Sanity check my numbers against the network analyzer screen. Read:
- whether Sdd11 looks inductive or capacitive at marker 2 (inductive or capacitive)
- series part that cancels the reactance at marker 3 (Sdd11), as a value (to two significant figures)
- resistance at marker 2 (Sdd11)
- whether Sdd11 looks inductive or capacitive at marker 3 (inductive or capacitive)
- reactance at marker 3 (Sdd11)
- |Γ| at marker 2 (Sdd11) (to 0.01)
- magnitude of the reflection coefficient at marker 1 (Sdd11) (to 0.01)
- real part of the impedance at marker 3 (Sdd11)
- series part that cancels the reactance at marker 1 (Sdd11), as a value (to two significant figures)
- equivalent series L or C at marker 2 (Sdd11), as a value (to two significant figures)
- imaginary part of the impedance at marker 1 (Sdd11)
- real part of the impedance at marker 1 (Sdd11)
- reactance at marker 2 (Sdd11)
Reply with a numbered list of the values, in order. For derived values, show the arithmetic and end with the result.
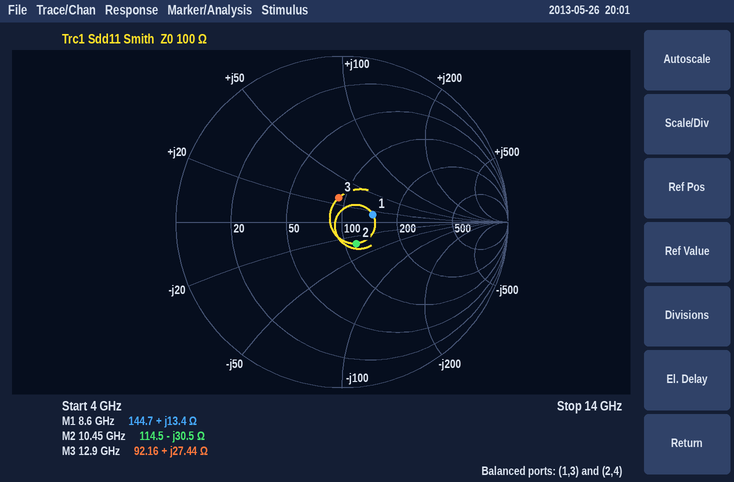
1. capacitive
2. C = 1/(2π × 12.9 GHz × 27.44 Ω) ≈ 450 fF
3. 114.5 Ω
4. inductive
5. +27.44 Ω
6. 0.16
7. 0.19
8. 92.16 Ω
9. C = 1/(2π × 8.6 GHz × 13.4 Ω) ≈ 1.4 pF
10. C = 1/(2π × 10.45 GHz × 30.5 Ω) ≈ 499 fF, so 500 fF to two significant figures
11. +13.4 Ω
12. 144.7 Ω
13. -30.5 Ω
